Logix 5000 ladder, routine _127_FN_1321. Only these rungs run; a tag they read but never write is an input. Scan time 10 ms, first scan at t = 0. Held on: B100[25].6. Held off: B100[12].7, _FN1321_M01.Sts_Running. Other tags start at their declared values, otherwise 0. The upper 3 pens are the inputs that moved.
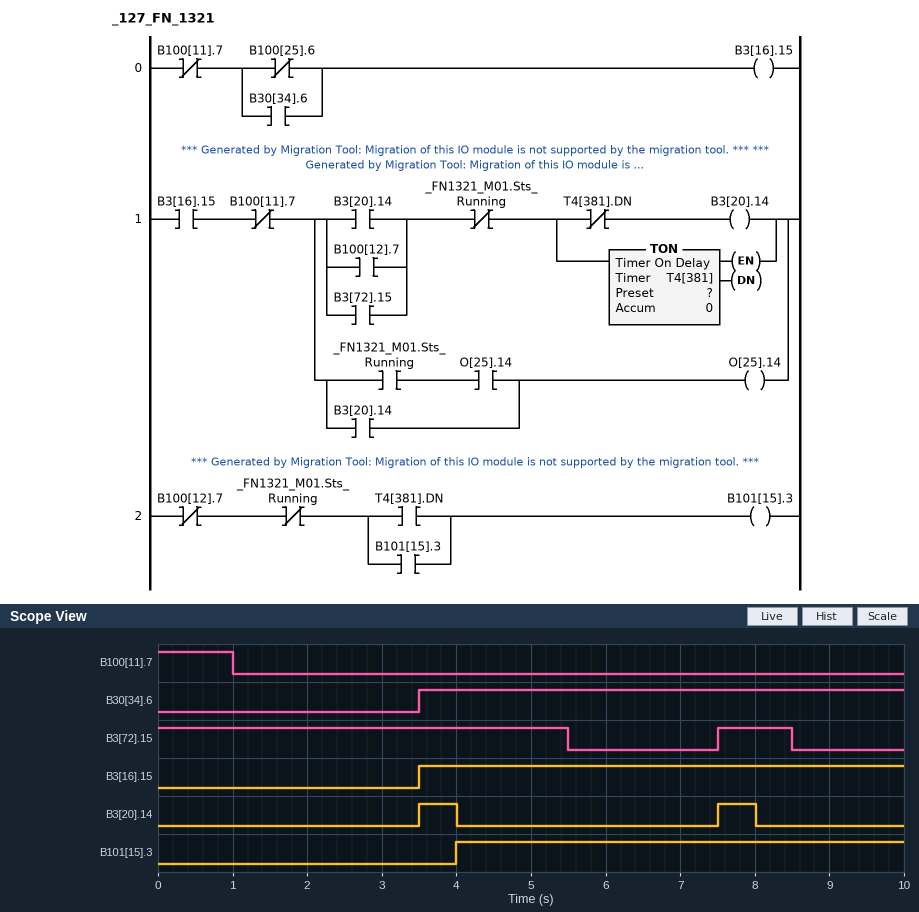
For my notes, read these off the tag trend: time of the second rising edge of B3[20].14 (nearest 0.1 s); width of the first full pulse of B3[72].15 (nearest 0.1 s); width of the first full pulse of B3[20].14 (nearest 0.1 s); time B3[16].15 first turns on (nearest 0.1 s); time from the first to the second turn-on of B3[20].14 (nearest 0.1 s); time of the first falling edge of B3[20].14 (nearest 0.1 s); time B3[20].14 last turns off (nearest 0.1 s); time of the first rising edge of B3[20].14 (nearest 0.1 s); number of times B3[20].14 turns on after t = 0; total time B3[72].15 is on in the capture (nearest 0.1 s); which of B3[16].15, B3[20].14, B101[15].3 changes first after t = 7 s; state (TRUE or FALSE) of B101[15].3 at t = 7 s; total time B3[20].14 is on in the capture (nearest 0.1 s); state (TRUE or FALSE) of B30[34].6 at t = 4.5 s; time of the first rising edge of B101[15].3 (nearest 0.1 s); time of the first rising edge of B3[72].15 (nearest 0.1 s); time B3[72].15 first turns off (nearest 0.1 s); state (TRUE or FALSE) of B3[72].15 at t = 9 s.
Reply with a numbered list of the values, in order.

1. 7.5 s
2. 1.0 s
3. 0.5 s
4. 3.5 s
5. 4.0 s
6. 4.0 s
7. 8.0 s
8. 3.5 s
9. 2
10. 6.5 s
11. B3[20].14
12. TRUE
13. 1.0 s
14. TRUE
15. 4.0 s
16. 7.5 s
17. 5.5 s
18. FALSE
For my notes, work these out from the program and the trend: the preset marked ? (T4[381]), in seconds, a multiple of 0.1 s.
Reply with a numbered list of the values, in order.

1. 0.5 s
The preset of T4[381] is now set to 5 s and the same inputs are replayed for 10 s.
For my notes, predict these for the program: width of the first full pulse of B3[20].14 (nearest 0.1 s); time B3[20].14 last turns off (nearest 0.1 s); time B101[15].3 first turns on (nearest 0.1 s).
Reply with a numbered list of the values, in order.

1. 5.0 s
2. 8.5 s
3. 8.5 s
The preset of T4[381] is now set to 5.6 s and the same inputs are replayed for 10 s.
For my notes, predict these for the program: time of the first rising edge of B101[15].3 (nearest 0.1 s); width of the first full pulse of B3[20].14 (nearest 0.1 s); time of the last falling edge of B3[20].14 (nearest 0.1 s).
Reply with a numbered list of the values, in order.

1. 9.1 s
2. 5.6 s
3. 9.1 s
